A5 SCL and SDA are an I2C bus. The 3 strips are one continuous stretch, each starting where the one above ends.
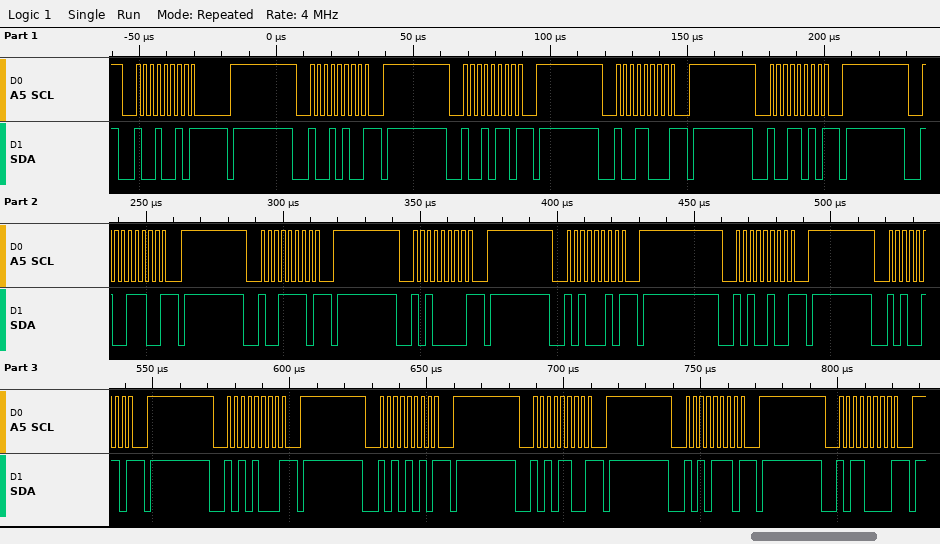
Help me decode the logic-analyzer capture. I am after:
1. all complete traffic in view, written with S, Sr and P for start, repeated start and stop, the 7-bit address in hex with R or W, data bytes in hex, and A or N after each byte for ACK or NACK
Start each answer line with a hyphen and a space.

- S 49W N P S 4AW N P S 4BW N P S 4CW N P S 4DW N P S 4EW N P S 4FW N P S 50W N P S 51W N P S 52W N P S 53W N P S 54W N P S 55W N P S 56W N P S 57W N P S 58W N P
